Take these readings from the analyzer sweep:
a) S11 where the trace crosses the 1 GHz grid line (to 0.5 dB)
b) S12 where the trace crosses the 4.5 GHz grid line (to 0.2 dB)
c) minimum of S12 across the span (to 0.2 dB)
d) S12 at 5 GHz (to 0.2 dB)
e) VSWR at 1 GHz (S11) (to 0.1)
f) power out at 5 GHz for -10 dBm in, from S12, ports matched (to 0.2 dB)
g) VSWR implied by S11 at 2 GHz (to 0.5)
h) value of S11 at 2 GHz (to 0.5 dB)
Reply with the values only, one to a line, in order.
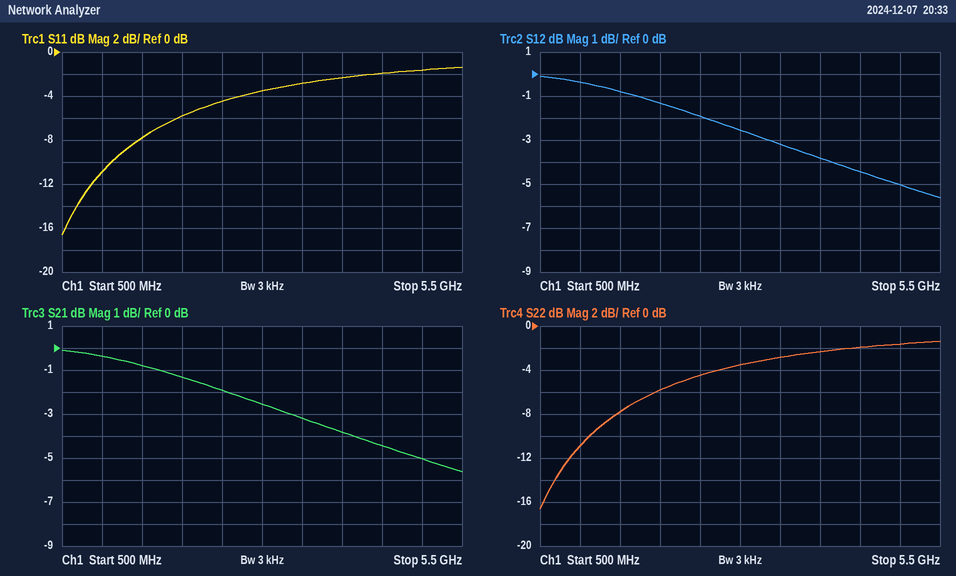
-11.0 dB
-4.4 dB
-5.6 dB
-5.0 dB
1.8
-15.0 dBm
3.0
-6.0 dB
